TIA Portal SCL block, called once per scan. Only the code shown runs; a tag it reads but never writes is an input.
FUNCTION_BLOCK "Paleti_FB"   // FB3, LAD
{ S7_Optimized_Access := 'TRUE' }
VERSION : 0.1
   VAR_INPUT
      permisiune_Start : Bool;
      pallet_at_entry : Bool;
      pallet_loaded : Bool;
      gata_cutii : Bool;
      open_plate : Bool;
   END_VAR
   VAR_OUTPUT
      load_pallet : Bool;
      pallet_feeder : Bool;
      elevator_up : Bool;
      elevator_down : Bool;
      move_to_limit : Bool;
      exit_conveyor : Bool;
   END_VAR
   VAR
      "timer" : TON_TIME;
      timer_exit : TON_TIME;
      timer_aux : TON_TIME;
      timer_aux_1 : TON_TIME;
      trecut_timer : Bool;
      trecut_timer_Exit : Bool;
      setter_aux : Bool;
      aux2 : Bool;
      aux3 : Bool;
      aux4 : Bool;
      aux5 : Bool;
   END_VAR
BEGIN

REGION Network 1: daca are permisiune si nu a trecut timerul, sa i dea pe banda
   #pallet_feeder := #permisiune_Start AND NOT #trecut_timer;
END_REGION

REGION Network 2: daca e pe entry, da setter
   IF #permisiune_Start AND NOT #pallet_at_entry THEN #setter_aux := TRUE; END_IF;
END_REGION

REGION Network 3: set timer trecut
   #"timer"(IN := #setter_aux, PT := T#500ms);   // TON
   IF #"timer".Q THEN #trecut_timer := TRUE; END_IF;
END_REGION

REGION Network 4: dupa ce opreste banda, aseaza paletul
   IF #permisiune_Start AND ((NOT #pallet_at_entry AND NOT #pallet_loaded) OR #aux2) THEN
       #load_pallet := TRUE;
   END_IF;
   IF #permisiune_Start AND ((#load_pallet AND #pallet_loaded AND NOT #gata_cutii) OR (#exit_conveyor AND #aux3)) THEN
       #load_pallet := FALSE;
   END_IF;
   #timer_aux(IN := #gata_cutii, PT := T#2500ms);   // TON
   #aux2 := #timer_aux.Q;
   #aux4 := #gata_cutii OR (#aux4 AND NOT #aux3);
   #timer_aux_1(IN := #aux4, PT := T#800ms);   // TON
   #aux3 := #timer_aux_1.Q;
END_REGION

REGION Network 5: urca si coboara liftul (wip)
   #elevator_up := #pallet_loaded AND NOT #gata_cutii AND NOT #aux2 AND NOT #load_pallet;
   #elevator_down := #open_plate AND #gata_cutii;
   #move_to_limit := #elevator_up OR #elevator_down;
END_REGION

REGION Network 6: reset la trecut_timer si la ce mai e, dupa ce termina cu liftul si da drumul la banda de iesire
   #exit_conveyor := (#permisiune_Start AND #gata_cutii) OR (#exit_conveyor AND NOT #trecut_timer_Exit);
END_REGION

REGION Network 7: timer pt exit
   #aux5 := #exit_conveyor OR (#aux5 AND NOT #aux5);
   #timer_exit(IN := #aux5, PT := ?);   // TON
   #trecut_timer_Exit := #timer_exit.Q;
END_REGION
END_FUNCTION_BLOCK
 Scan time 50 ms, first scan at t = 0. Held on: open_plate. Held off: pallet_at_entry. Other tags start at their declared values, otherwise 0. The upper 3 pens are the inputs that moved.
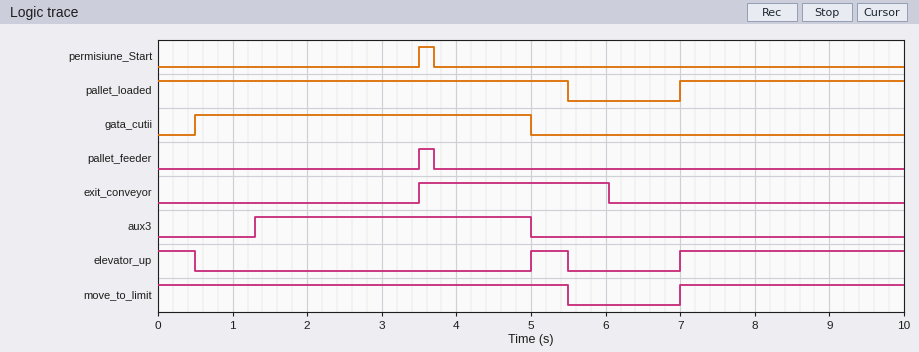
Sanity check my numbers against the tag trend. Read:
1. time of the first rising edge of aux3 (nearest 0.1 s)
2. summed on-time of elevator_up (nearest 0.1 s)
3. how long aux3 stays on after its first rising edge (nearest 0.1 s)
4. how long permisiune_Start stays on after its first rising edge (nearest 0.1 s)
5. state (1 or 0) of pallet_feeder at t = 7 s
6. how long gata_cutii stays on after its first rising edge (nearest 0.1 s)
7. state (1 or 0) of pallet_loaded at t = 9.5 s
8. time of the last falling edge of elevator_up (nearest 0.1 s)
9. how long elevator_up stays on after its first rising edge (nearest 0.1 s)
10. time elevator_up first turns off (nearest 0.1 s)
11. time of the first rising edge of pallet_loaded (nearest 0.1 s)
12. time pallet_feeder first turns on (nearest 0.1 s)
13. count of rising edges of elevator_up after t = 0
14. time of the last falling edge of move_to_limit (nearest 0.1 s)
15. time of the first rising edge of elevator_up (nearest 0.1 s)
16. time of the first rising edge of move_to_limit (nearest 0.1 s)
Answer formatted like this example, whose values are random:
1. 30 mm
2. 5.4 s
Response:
1. 1.3 s
2. 4.0 s
3. 3.7 s
4. 0.2 s
5. 0
6. 4.5 s
7. 1
8. 5.5 s
9. 0.5 s
10. 0.5 s
11. 7.0 s
12. 3.5 s
13. 2
14. 5.5 s
15. 5.0 s
16. 7.0 s
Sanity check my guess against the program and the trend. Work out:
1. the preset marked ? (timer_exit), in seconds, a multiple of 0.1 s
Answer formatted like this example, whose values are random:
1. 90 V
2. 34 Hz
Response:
1. 2.5 s
